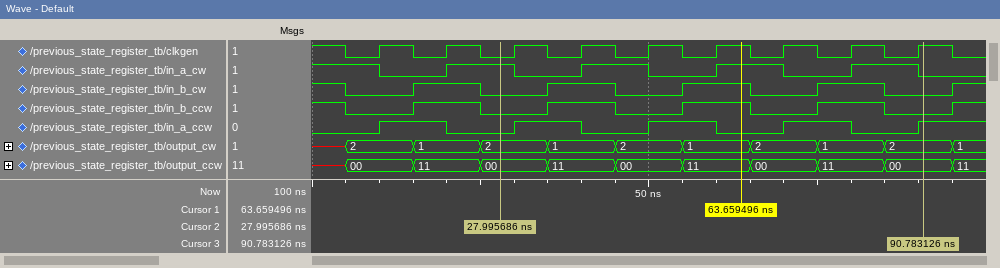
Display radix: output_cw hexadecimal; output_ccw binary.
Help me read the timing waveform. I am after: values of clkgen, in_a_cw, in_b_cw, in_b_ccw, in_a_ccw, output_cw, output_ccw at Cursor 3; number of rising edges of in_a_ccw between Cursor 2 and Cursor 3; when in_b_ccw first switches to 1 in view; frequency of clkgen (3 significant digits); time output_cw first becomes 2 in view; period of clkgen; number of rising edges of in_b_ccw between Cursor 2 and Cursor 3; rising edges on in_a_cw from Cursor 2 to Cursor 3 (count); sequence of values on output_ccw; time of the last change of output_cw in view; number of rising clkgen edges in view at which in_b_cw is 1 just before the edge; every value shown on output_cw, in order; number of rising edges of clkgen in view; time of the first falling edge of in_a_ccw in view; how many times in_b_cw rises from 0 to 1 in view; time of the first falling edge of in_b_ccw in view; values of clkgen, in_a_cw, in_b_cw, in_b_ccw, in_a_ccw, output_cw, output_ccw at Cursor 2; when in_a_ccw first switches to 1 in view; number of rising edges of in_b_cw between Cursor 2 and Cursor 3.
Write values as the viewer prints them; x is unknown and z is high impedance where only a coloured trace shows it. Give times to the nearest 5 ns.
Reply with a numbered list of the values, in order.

1. clkgen=1, in_a_cw=0, in_b_cw=0, in_b_ccw=0, in_a_ccw=1, output_cw=2, output_ccw=00
2. 4
3. 15 ns
4. 100 MHz
5. 5 ns
6. 10 ns
7. 3
8. 3
9. x, 00, 11, 00, 11, 00, 11, 00, 11, 00, 11
10. 95 ns
11. 4
12. x, 2, 1, 2, 1, 2, 1, 2, 1, 2, 1
13. 9
14. 20 ns
15. 5
16. 5 ns
17. clkgen=0, in_a_cw=1, in_b_cw=0, in_b_ccw=0, in_a_ccw=0, output_cw=2, output_ccw=00
18. 10 ns
19. 3
